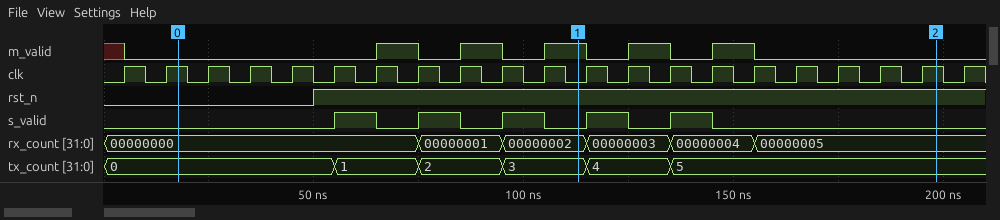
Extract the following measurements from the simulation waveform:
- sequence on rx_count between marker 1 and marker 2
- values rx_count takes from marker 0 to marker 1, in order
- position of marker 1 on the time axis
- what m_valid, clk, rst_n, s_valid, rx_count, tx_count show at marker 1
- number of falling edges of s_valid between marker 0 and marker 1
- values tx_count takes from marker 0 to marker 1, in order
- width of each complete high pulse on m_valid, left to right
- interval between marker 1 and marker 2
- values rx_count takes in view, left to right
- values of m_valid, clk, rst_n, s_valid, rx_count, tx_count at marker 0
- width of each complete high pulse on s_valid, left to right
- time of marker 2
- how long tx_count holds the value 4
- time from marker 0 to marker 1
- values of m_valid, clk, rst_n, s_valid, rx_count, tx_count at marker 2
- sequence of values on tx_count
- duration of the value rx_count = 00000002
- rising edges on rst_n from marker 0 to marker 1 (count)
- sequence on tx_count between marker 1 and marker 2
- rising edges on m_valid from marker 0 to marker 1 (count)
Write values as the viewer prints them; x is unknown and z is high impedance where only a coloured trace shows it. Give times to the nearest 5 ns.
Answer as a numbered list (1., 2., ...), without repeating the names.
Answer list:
1. 00000002, 00000003, 00000004, 00000005
2. 00000000, 00000001, 00000002
3. 115 ns
4. m_valid=1, clk=0, rst_n=1, s_valid=0, rx_count=00000002, tx_count=3
5. 3
6. 0, 1, 2, 3
7. 10 ns, 10 ns, 10 ns, 10 ns, 10 ns
8. 85 ns
9. 00000000, 00000001, 00000002, 00000003, 00000004, 00000005
10. m_valid=0, clk=1, rst_n=0, s_valid=0, rx_count=00000000, tx_count=0
11. 10 ns, 10 ns, 10 ns, 10 ns, 10 ns
12. 200 ns
13. 20 ns
14. 95 ns
15. m_valid=0, clk=1, rst_n=1, s_valid=0, rx_count=00000005, tx_count=5
16. 0, 1, 2, 3, 4, 5
17. 20 ns
18. 1
19. 3, 4, 5
20. 3
